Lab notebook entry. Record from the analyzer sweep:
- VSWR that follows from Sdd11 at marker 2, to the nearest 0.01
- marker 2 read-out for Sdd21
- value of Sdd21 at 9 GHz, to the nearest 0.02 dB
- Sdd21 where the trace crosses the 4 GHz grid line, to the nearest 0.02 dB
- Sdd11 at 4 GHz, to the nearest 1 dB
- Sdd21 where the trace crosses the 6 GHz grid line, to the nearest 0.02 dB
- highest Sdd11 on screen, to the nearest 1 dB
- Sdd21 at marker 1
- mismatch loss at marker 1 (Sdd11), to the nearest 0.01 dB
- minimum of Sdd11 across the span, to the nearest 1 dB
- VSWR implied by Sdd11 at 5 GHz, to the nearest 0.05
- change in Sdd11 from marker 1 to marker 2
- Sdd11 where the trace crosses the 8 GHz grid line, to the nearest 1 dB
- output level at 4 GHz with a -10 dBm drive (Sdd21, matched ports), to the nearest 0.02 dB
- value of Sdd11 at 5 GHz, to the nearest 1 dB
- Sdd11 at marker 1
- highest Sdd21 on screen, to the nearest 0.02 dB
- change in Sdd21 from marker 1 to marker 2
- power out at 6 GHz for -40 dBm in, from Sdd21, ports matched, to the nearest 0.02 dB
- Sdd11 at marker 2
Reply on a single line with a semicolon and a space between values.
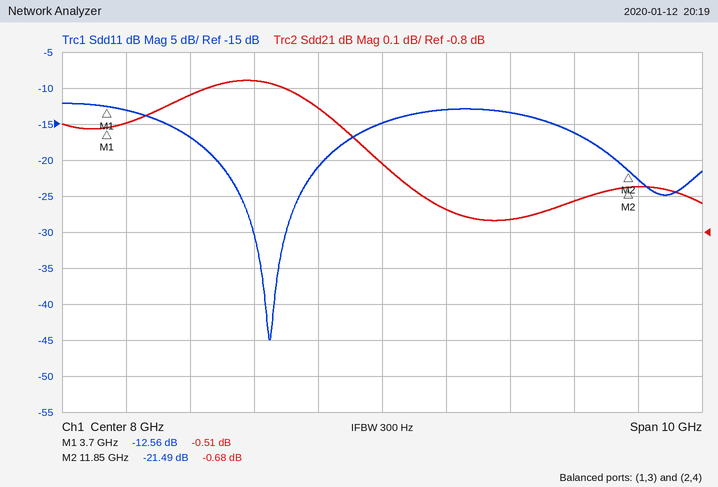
1.18; -0.68 dB; -0.74 dB; -0.50 dB; -13 dB; -0.38 dB; -12 dB; -0.51 dB; 0.25 dB; -45 dB; 1.35; -8.93 dB; -15 dB; -10.50 dBm; -17 dB; -12.56 dB; -0.38 dB; -0.17 dB; -40.38 dBm; -21.49 dB
